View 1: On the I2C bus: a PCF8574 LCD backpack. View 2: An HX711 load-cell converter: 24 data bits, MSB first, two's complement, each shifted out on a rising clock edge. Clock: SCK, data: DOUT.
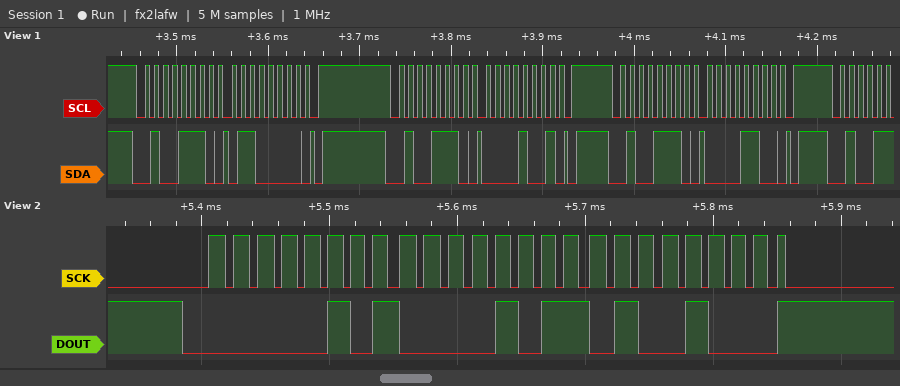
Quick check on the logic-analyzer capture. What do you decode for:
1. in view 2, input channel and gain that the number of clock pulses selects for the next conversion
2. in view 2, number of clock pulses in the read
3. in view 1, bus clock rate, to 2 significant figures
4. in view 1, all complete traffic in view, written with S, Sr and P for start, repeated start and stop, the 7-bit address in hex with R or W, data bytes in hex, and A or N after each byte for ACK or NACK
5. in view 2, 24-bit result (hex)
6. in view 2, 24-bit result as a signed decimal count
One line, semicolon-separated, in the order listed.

channel A, gain 128; 25; 100 kHz; S 27W A 60 A P S 27W A 09 A P S 27W A 0C A P; 0x050B48; 330568
